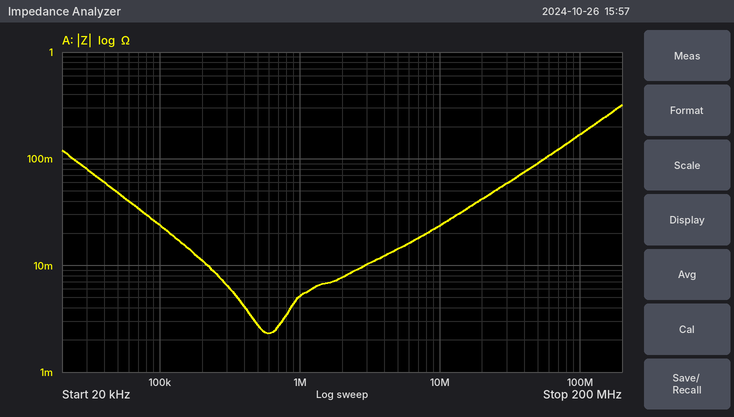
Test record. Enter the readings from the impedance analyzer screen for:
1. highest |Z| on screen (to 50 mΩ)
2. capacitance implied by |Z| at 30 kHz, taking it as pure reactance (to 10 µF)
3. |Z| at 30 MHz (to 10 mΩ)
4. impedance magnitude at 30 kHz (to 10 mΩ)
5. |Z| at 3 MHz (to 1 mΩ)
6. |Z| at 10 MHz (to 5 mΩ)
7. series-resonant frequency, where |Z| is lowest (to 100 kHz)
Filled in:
300 mΩ
70 µF
60 mΩ
80 mΩ
10 mΩ
25 mΩ
600 kHz
